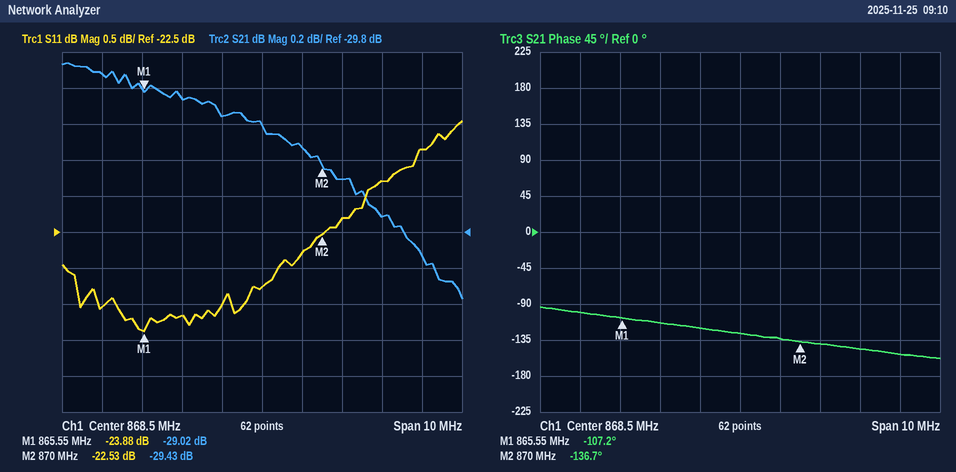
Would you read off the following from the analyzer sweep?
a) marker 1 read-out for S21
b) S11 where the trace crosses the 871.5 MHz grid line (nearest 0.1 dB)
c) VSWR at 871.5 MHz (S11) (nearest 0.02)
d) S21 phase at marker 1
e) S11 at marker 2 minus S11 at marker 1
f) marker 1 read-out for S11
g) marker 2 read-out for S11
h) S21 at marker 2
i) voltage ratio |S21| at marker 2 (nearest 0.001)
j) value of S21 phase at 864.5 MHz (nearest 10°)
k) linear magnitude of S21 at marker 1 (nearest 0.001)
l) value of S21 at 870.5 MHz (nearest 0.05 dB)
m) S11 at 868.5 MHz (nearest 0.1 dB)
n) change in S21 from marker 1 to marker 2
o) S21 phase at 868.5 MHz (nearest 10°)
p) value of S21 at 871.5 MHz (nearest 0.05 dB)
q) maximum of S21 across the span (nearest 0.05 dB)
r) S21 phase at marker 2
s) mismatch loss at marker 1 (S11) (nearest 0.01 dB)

-29.02 dB
-21.8 dB
1.18
-107.2°
1.35 dB
-23.88 dB
-22.53 dB
-29.43 dB
0.034
-100°
0.035
-29.50 dB
-23.3 dB
-0.41 dB
-130°
-29.70 dB
-28.85 dB
-136.7°
0.02 dB
